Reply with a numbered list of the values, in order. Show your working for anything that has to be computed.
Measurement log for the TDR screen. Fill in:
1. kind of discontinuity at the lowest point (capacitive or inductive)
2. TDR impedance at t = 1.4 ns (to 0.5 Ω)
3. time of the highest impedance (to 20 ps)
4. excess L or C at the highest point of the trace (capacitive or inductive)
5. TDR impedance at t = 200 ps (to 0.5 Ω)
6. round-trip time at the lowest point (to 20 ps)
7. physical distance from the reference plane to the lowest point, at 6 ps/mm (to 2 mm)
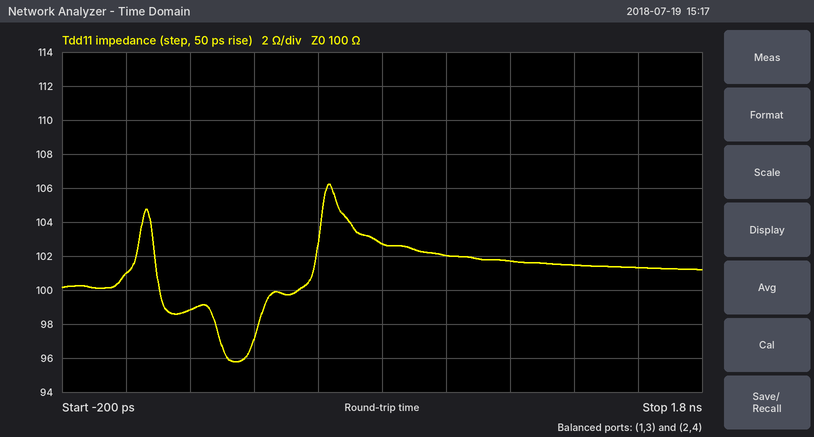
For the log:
1. capacitive
2. 101.5 Ω
3. 640 ps
4. inductive
5. 99.0 Ω
6. 340 ps
7. 340 ps / 2 / 6 ps/mm ≈ 28 mm
